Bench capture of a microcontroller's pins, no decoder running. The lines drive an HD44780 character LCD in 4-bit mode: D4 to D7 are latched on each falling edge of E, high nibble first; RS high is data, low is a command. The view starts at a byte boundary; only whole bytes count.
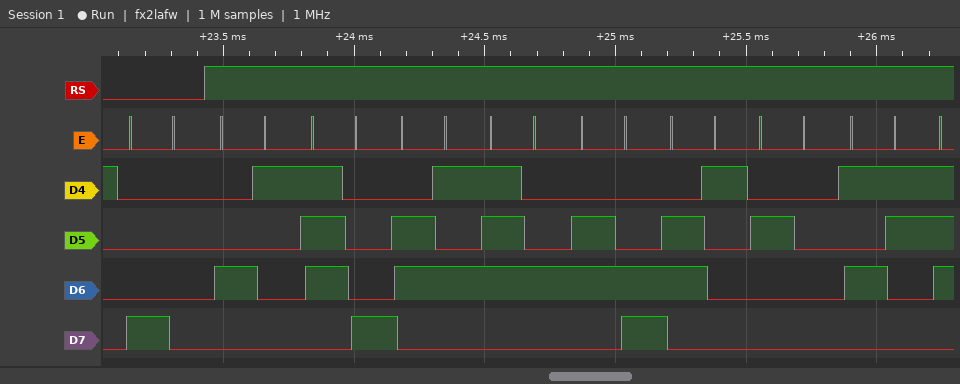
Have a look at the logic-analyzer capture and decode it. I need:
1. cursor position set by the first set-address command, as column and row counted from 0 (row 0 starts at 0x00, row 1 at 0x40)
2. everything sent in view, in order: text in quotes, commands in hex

column 0, row 0
0x80 "Axetla S"
